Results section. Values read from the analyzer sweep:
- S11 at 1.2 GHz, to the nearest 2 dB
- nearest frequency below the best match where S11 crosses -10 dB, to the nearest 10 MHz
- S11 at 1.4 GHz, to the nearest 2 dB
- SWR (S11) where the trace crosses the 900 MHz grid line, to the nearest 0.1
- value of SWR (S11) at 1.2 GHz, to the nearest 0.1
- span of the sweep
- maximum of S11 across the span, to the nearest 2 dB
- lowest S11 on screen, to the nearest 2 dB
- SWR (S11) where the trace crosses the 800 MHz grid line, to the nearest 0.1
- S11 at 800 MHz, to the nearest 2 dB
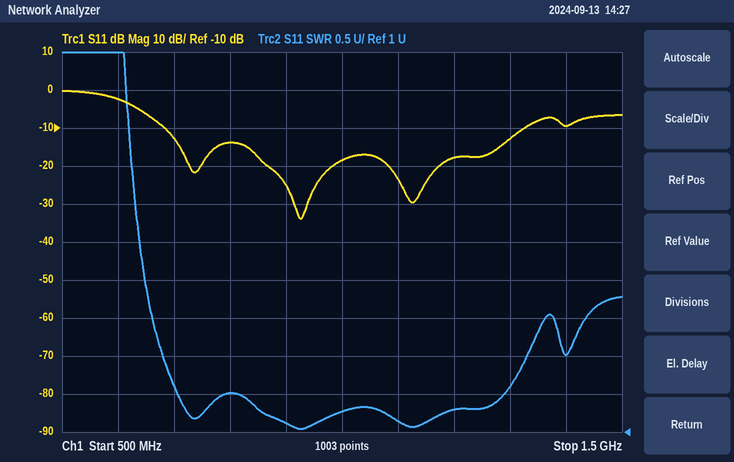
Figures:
-18 dB
680 MHz
-10 dB
1.1
1.3
1 GHz
0 dB
-34 dB
1.5
-14 dB
